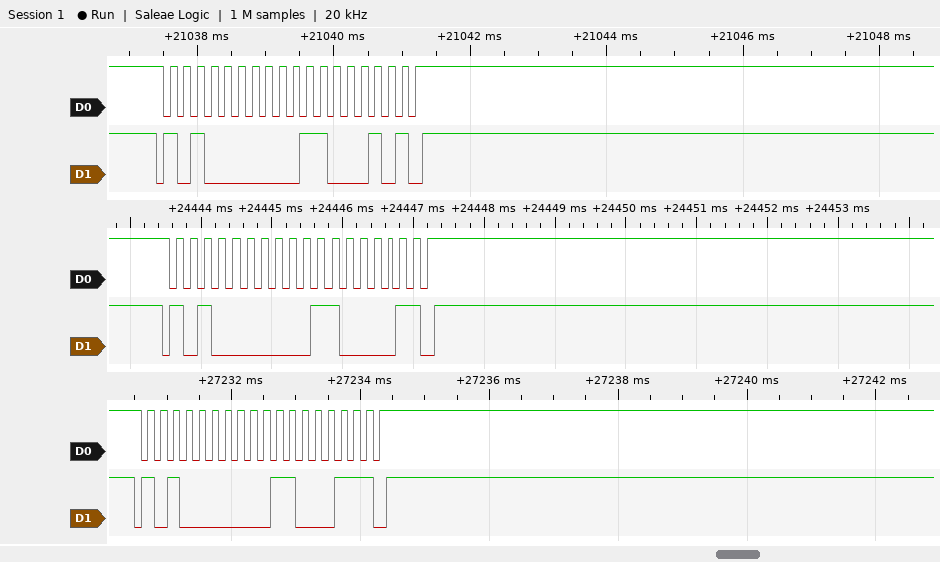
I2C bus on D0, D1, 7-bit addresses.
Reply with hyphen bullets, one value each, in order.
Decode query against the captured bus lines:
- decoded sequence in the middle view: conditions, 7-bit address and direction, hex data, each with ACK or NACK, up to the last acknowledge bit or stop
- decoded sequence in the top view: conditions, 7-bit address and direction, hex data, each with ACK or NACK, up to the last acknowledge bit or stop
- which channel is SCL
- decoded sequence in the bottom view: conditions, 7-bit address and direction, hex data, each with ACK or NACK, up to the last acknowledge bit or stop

- start, address 50 write ACK, 61 NACK, stop
- start, address 50 write ACK, 62 NACK, stop
- D0
- start, address 50 write ACK, 63 NACK, stop
